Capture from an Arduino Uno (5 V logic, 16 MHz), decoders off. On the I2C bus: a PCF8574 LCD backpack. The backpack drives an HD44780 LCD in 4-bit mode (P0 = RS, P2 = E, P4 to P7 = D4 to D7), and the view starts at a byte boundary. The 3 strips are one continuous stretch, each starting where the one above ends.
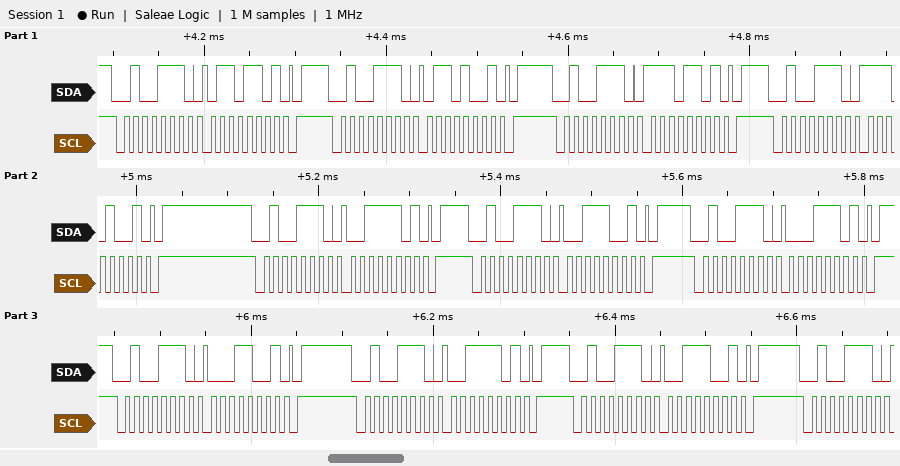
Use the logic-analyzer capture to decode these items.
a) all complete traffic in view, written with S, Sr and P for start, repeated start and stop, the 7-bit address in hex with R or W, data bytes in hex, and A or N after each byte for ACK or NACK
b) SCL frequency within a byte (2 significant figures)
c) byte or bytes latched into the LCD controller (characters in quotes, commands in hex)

S 27W A 6D A P S 27W A 69 A P S 27W A ED A P S 27W A E9 A P S 27W A 3D A P S 27W A 39 A P S 27W A 1D A P S 27W A 19 A P S 27W A 3D A P S 27W A 39 A P S 27W A
100 kHz
'n' '1'
